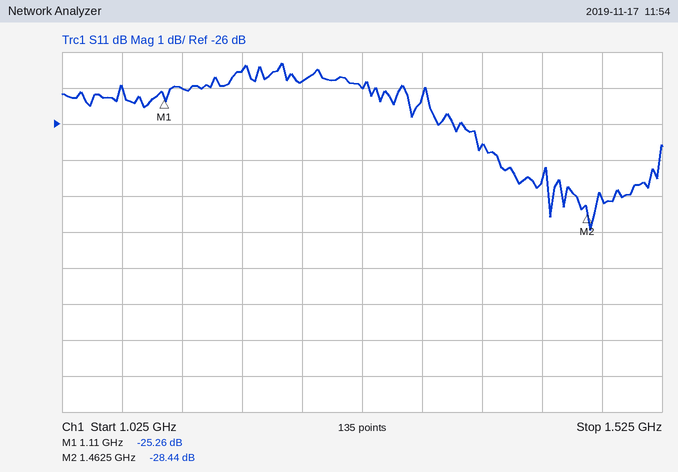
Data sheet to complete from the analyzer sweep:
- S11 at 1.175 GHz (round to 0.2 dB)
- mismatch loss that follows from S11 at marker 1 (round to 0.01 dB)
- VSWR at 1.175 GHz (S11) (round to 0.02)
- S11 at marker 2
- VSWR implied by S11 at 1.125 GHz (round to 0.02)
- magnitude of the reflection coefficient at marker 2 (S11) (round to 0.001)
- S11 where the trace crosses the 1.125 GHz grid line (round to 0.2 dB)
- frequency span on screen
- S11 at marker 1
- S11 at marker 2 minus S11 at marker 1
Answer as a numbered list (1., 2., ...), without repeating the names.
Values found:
1. -24.6 dB
2. 0.01 dB
3. 1.12
4. -28.44 dB
5. 1.12
6. 0.038
7. -25.0 dB
8. 500 MHz
9. -25.26 dB
10. -3.18 dB
